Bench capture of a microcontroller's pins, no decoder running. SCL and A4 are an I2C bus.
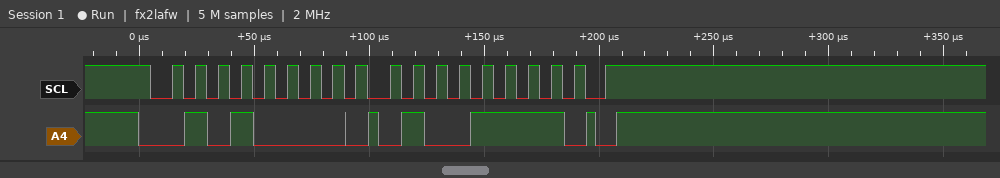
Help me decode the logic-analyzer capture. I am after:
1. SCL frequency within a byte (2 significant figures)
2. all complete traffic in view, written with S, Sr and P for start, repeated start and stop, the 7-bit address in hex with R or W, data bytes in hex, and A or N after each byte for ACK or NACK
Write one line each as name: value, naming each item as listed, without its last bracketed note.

SCL frequency within a byte: 100 kHz
all complete traffic in view, written with S, Sr and P for start, repeated start and stop, the 7-bit address in hex with R or W, data bytes in hex, and A or N after each byte for ACK or NACK: S 28W A 4F A P
